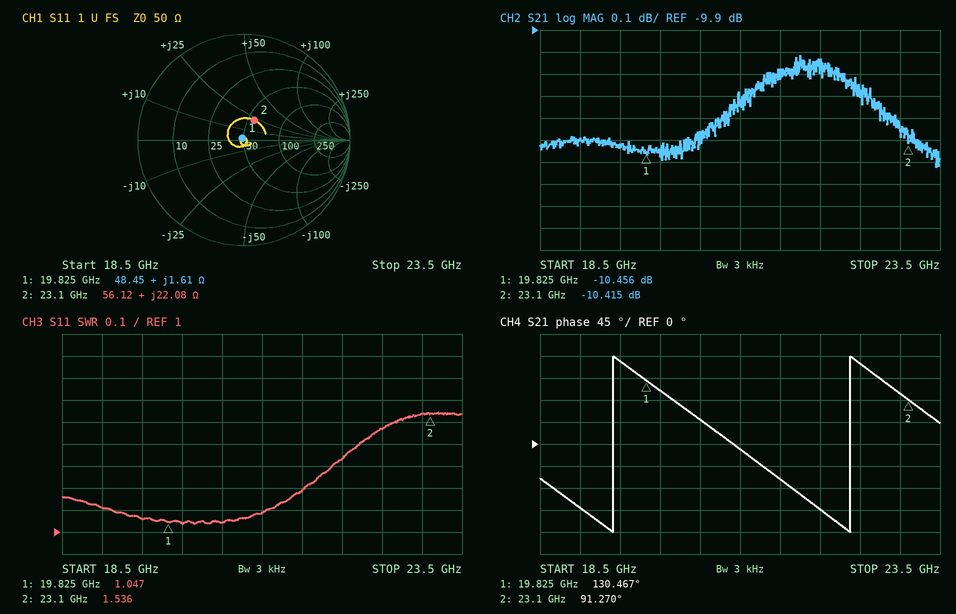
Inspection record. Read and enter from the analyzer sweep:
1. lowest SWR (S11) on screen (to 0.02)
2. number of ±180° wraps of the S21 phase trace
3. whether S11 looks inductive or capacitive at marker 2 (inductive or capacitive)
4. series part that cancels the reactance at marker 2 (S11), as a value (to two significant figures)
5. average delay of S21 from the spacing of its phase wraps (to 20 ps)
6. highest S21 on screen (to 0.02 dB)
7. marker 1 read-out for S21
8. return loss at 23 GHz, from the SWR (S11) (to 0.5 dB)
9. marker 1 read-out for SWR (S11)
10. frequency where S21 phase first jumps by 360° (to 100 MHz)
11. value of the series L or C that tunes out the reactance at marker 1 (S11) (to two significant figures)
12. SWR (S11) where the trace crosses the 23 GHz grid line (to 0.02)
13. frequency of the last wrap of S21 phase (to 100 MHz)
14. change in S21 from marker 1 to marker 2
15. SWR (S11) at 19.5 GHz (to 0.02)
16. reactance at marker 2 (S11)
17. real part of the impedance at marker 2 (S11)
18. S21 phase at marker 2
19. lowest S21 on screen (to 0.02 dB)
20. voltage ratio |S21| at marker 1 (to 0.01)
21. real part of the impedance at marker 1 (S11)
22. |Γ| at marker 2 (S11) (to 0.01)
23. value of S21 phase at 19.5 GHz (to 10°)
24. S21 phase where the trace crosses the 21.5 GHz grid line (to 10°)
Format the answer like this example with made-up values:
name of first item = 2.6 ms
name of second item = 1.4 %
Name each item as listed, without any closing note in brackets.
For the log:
lowest SWR (S11) on screen = 1.04
number of ±180° wraps of the S21 phase trace = 2
whether S11 looks inductive or capacitive at marker 2 = inductive
series part that cancels the reactance at marker 2 (S11), as a value = 310 fF
average delay of S21 from the spacing of its phase wraps = 340 ps
highest S21 on screen = -10.02 dB
marker 1 read-out for S21 = -10.456 dB
return loss at 23 GHz, from the SWR (S11) = 13.5 dB
marker 1 read-out for SWR = 1.047
frequency where S21 phase first jumps by 360° = 19.4 GHz
value of the series L or C that tunes out the reactance at marker 1 (S11) = 5.0 pF
SWR (S11) where the trace crosses the 23 GHz grid line = 1.54
frequency of the last wrap of S21 phase = 22.4 GHz
change in S21 from marker 1 to marker 2 = 0.041 dB
SWR (S11) at 19.5 GHz = 1.06
reactance at marker 2 = +22.08 Ω
real part of the impedance at marker 2 = 56.12 Ω
S21 phase at marker 2 = 91.270°
lowest S21 on screen = -10.52 dB
voltage ratio |S21| at marker 1 = 0.30
real part of the impedance at marker 1 = 48.45 Ω
|Γ| at marker 2 (S11) = 0.21
value of S21 phase at 19.5 GHz = 170°
S21 phase where the trace crosses the 21.5 GHz grid line = -70°
